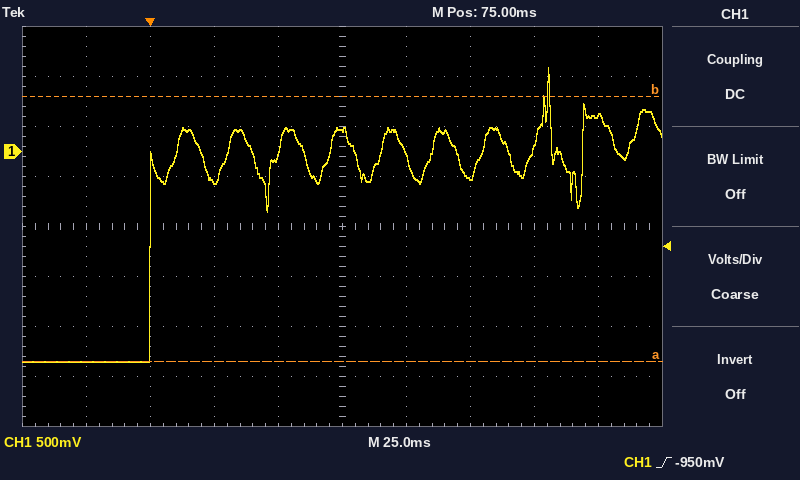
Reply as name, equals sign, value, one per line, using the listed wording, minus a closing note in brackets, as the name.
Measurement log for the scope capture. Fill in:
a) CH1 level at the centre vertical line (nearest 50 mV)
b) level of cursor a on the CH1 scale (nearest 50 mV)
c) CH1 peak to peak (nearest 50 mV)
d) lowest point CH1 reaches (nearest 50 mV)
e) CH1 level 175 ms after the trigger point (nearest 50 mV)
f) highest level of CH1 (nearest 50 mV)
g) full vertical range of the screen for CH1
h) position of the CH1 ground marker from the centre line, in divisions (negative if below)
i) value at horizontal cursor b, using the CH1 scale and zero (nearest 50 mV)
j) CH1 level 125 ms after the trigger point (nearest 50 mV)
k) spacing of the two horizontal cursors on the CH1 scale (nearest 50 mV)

CH1 level at the centre vertical line = 200 mV
level of cursor a on the CH1 scale = -2.10 V
CH1 peak to peak = 2.95 V
lowest point CH1 reaches = -2.10 V
CH1 level 175 ms after the trigger point = 350 mV
highest level of CH1 = 850 mV
full vertical range of the screen for CH1 = 4 V
position of the CH1 ground marker from the centre line, in divisions = +1.5 div
value at horizontal cursor b, using the CH1 scale and zero = 550 mV
CH1 level 125 ms after the trigger point = -250 mV
spacing of the two horizontal cursors on the CH1 scale = 2.65 V
